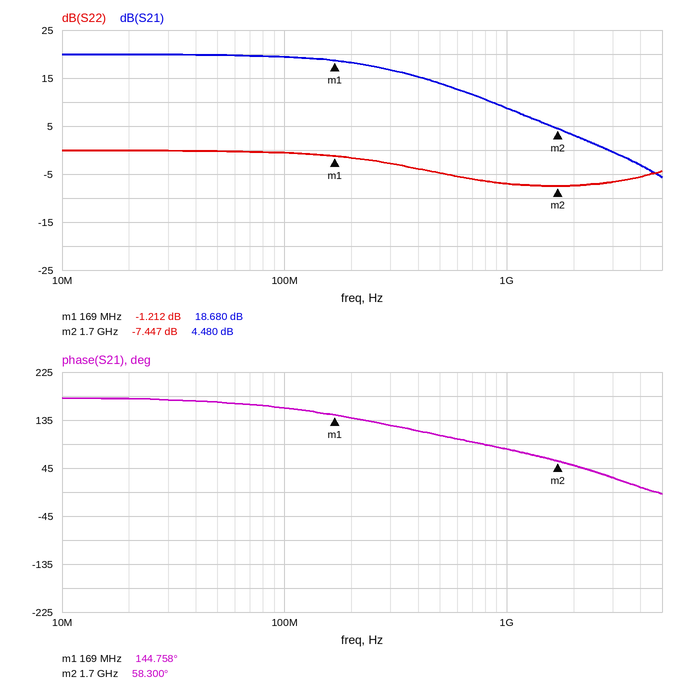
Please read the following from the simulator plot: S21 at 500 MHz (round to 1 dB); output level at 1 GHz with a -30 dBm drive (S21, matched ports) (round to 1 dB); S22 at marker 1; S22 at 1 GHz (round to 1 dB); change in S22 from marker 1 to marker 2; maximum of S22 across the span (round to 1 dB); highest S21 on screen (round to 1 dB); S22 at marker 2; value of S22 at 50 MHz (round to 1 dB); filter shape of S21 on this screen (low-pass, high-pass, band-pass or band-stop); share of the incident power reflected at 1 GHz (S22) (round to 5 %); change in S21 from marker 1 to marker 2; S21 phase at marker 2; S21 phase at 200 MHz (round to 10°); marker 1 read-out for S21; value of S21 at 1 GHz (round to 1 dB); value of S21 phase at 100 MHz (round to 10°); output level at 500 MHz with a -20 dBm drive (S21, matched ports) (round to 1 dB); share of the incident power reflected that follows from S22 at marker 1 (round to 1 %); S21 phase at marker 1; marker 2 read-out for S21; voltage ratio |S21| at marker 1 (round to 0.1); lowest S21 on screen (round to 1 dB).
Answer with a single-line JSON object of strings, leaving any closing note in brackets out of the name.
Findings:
{"S21 at 500 MHz": "14 dB", "output level at 1 GHz with a -30 dBm drive (S21, matched ports)": "-21 dBm", "S22 at marker 1": "-1.212 dB", "S22 at 1 GHz": "-7 dB", "change in S22 from marker 1 to marker 2": "-6.235 dB", "maximum of S22 across the span": "0 dB", "highest S21 on screen": "20 dB", "S22 at marker 2": "-7.447 dB", "value of S22 at 50 MHz": "0 dB", "filter shape of S21 on this screen": "low-pass", "share of the incident power reflected at 1 GHz (S22)": "20 %", "change in S21 from marker 1 to marker 2": "-14.200 dB", "S21 phase at marker 2": "58.300°", "S21 phase at 200 MHz": "140°", "marker 1 read-out for S21": "18.680 dB", "value of S21 at 1 GHz": "9 dB", "value of S21 phase at 100 MHz": "160°", "output level at 500 MHz with a -20 dBm drive (S21, matched ports)": "-6 dBm", "share of the incident power reflected that follows from S22 at marker 1": "76 %", "S21 phase at marker 1": "144.758°", "marker 2 read-out for S21": "4.480 dB", "voltage ratio |S21| at marker 1": "8.6", "lowest S21 on screen": "-6 dB"}
